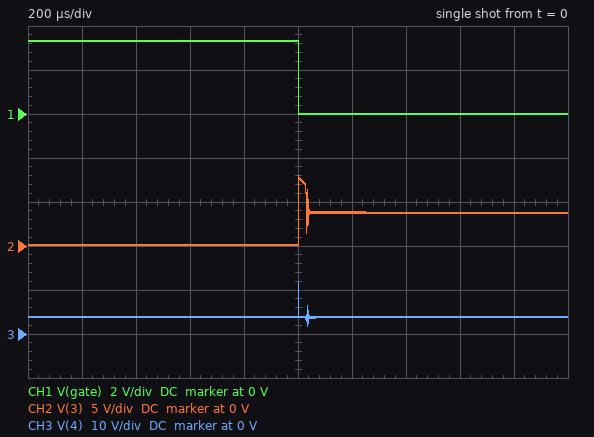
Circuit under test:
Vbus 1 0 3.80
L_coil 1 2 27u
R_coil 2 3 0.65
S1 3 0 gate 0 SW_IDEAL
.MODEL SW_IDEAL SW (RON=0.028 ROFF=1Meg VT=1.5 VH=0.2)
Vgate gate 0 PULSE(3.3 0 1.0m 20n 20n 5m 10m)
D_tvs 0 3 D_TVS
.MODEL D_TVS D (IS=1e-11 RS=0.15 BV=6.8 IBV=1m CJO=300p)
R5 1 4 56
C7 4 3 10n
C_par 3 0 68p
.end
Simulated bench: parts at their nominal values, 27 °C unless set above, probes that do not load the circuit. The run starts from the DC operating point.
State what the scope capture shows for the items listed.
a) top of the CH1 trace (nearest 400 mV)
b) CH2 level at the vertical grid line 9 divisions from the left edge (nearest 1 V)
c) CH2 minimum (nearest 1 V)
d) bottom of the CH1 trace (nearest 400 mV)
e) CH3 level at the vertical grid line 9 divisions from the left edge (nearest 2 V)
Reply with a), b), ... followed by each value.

a) 3.2 V
b) 4 V
c) 0 V
d) 0 V
e) 4 V
